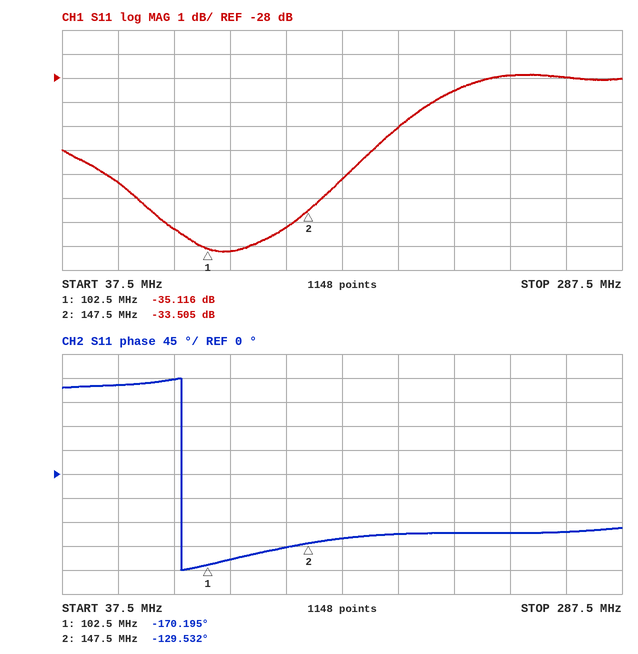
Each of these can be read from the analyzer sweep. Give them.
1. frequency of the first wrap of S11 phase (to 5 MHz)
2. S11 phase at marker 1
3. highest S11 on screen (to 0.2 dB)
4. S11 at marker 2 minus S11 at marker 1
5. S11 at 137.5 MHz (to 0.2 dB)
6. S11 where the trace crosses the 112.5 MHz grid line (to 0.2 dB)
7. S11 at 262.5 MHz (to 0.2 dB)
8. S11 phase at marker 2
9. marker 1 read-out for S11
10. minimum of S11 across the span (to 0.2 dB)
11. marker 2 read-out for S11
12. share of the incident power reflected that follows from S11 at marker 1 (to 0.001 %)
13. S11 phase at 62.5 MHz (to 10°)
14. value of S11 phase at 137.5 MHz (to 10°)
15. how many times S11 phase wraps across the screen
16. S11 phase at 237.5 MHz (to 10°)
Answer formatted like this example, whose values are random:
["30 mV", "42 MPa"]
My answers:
["90 MHz", "-170.195°", "-27.8 dB", "1.611 dB", "-34.2 dB", "-35.2 dB", "-28.0 dB", "-129.532°", "-35.116 dB", "-35.2 dB", "-33.505 dB", "0.031 %", "170°", "-140°", "1", "-110°"]
